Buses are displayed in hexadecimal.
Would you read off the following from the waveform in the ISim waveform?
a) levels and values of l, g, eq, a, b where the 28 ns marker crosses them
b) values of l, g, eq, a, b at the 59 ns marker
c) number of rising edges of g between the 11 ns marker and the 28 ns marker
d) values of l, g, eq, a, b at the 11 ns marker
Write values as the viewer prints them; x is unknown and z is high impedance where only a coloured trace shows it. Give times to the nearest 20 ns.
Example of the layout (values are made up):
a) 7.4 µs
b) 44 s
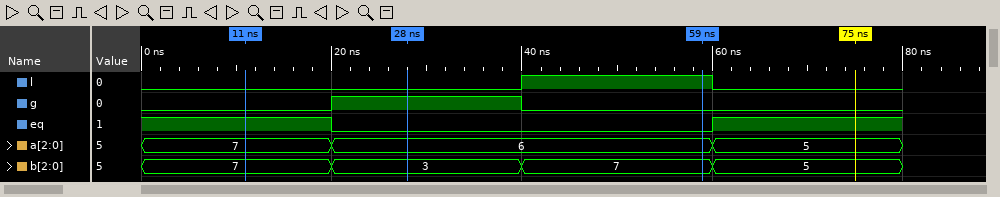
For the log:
a) l=0, g=1, eq=0, a=6, b=3
b) l=1, g=0, eq=0, a=6, b=7
c) 1
d) l=0, g=0, eq=1, a=7, b=7
